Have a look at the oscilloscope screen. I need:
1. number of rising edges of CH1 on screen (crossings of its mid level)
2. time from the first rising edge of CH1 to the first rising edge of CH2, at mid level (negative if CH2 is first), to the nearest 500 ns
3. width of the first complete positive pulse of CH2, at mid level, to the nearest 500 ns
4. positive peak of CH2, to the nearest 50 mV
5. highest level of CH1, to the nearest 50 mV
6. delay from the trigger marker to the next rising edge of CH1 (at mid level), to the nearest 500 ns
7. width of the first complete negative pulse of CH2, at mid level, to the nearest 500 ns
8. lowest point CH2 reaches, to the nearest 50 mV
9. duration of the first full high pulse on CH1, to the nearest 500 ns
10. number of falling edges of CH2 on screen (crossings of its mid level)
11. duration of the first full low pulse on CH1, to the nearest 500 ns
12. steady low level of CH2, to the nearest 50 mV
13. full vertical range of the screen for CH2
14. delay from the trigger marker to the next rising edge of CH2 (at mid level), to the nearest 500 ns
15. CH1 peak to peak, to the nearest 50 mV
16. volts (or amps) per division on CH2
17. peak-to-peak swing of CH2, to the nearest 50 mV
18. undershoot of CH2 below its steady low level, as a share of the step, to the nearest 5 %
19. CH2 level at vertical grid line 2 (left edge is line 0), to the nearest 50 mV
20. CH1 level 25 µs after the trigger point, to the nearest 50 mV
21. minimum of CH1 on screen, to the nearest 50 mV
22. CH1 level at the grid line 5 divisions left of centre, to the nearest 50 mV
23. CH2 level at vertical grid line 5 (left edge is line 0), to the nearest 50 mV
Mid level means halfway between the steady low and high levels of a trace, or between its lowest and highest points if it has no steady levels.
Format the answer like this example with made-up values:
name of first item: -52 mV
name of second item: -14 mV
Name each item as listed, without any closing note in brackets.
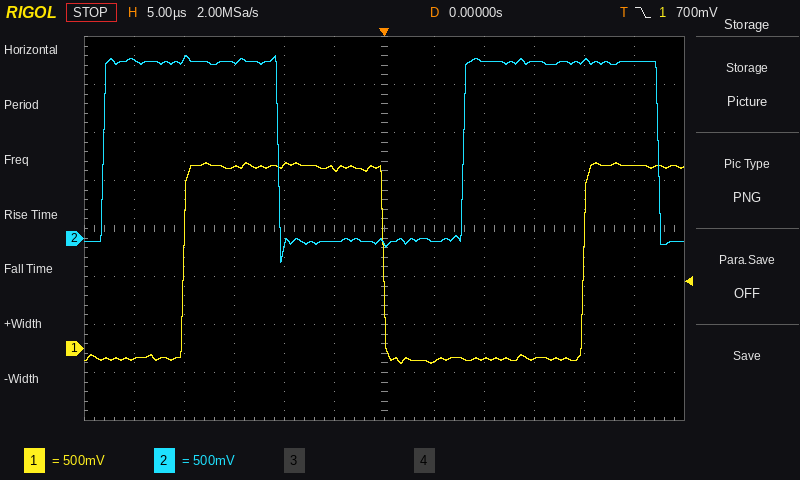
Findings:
number of rising edges of CH1 on screen: 2
time from the first rising edge of CH1 to the first rising edge of CH2, at mid level (negative if CH2 is first), to the nearest 500 ns: -8.0 µs
width of the first complete positive pulse of CH2, at mid level, to the nearest 500 ns: 17.5 µs
positive peak of CH2, to the nearest 50 mV: 1.90 V
highest level of CH1, to the nearest 50 mV: 1.95 V
delay from the trigger marker to the next rising edge of CH1 (at mid level), to the nearest 500 ns: 20.0 µs
width of the first complete negative pulse of CH2, at mid level, to the nearest 500 ns: 18.5 µs
lowest point CH2 reaches, to the nearest 50 mV: -250 mV
duration of the first full high pulse on CH1, to the nearest 500 ns: 20.0 µs
number of falling edges of CH2 on screen: 2
duration of the first full low pulse on CH1, to the nearest 500 ns: 20.0 µs
steady low level of CH2, to the nearest 50 mV: -50 mV
full vertical range of the screen for CH2: 4 V
delay from the trigger marker to the next rising edge of CH2 (at mid level), to the nearest 500 ns: 8.0 µs
CH1 peak to peak, to the nearest 50 mV: 2.10 V
volts (or amps) per division on CH2: 500 mV
peak-to-peak swing of CH2, to the nearest 50 mV: 2.15 V
undershoot of CH2 below its steady low level, as a share of the step, to the nearest 5 %: 10 %
CH2 level at vertical grid line 2 (left edge is line 0), to the nearest 50 mV: 1.85 V
CH1 level 25 µs after the trigger point, to the nearest 50 mV: 1.90 V
minimum of CH1 on screen, to the nearest 50 mV: -150 mV
CH1 level at the grid line 5 divisions left of centre, to the nearest 50 mV: -100 mV
CH2 level at vertical grid line 5 (left edge is line 0), to the nearest 50 mV: -50 mV
